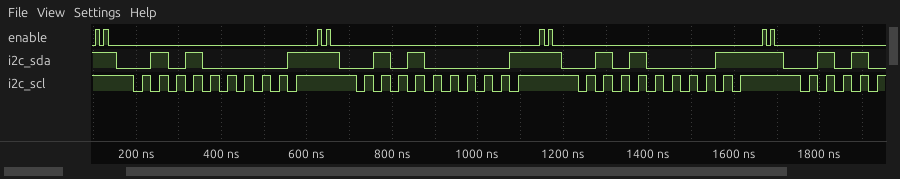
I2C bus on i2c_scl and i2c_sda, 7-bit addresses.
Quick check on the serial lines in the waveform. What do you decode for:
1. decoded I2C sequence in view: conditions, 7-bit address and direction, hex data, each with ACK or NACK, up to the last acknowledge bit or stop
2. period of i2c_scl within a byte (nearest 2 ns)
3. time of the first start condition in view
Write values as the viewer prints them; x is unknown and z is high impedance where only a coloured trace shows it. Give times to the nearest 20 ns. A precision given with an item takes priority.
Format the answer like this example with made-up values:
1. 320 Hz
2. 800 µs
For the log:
1. start, address 28 write ACK, repeated start, address 28 write ACK, repeated start, address 28 write NACK
2. 40 ns
3. 160 ns
